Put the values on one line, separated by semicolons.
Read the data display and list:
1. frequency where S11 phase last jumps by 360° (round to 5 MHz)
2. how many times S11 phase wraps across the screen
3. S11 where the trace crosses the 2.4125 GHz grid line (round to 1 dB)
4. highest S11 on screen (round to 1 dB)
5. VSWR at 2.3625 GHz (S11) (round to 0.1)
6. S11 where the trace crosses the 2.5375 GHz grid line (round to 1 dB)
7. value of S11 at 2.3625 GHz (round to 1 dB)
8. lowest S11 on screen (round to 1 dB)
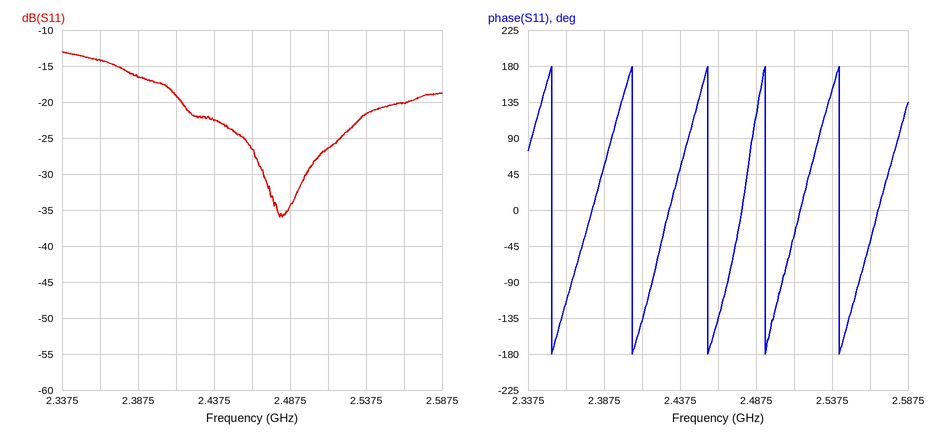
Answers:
2.540 GHz; 5; -19 dB; -13 dB; 1.5; -22 dB; -14 dB; -36 dB
